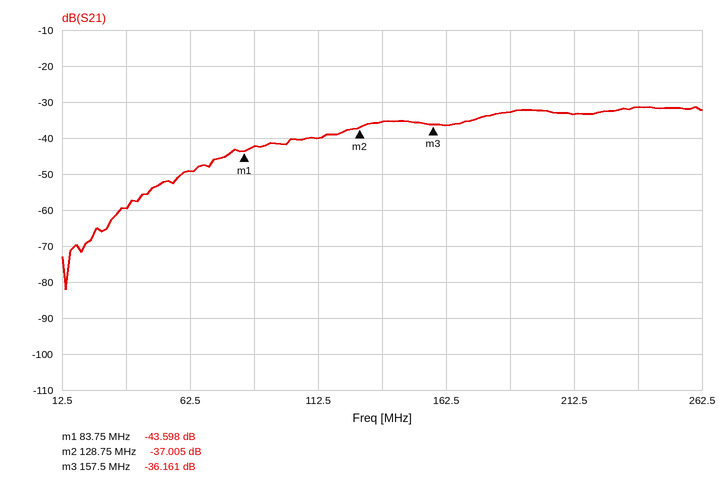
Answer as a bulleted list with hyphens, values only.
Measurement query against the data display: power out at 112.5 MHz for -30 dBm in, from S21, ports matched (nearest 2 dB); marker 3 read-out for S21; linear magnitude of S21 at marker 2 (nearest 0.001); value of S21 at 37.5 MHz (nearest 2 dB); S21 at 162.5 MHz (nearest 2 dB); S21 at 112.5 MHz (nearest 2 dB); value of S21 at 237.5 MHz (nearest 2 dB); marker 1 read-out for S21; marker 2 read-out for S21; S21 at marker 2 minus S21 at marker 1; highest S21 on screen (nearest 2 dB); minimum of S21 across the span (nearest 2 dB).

- -70 dBm
- -36.161 dB
- 0.014
- -60 dB
- -36 dB
- -40 dB
- -32 dB
- -43.598 dB
- -37.005 dB
- 6.593 dB
- -32 dB
- -82 dB
